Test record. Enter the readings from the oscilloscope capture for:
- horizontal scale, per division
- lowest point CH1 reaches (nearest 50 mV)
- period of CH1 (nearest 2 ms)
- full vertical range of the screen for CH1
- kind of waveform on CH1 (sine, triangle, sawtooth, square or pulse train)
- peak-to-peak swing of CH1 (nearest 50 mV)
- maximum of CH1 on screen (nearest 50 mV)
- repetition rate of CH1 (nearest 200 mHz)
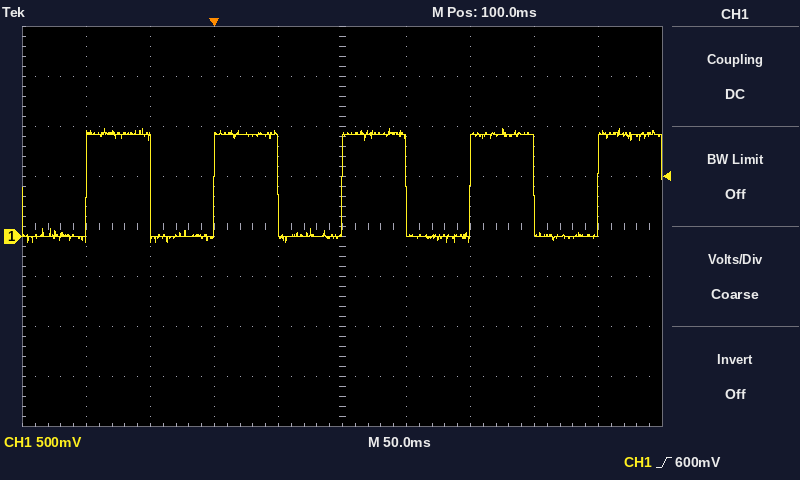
50 ms
-50 mV
100 ms
4 V
square
1.15 V
1.10 V
10.0 Hz
